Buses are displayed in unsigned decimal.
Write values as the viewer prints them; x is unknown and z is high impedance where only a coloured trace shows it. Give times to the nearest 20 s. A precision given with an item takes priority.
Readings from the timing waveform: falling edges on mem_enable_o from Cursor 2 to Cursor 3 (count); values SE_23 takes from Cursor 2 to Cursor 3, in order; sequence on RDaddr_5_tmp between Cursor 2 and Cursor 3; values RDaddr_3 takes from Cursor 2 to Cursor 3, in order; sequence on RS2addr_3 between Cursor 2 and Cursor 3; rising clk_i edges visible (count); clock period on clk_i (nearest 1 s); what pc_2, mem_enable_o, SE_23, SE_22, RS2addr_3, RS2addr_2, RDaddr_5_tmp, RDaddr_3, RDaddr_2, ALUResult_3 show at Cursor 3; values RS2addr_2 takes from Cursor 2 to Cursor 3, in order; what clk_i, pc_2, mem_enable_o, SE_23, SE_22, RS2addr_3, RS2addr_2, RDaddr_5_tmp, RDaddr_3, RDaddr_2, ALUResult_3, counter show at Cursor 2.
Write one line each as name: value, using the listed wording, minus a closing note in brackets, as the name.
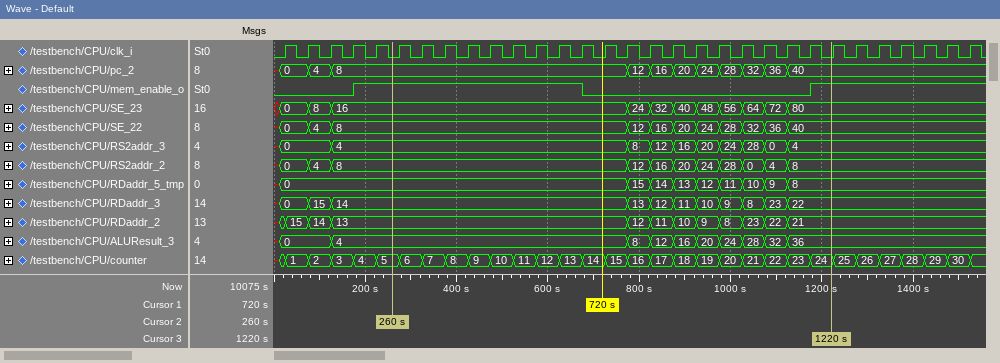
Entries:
falling edges on mem_enable_o from Cursor 2 to Cursor 3: 1
values SE_23 takes from Cursor 2 to Cursor 3, in order: 16, 24, 32, 40, 48, 56, 64, 72, 80
sequence on RDaddr_5_tmp between Cursor 2 and Cursor 3: 0, 15, 14, 13, 12, 11, 10, 9, 8
values RDaddr_3 takes from Cursor 2 to Cursor 3, in order: 14, 13, 12, 11, 10, 9, 8, 23, 22
sequence on RS2addr_3 between Cursor 2 and Cursor 3: 4, 8, 12, 16, 20, 24, 28, 0, 4
rising clk_i edges visible: 31
clock period on clk_i: 50 s
what pc_2, mem_enable_o, SE_23, SE_22, RS2addr_3, RS2addr_2, RDaddr_5_tmp, RDaddr_3, RDaddr_2, ALUResult_3 show at Cursor 3: pc_2=40, mem_enable_o=1, SE_23=80, SE_22=40, RS2addr_3=4, RS2addr_2=8, RDaddr_5_tmp=8, RDaddr_3=22, RDaddr_2=21, ALUResult_3=36
values RS2addr_2 takes from Cursor 2 to Cursor 3, in order: 8, 12, 16, 20, 24, 28, 0, 4, 8
what clk_i, pc_2, mem_enable_o, SE_23, SE_22, RS2addr_3, RS2addr_2, RDaddr_5_tmp, RDaddr_3, RDaddr_2, ALUResult_3, counter show at Cursor 2: clk_i=0, pc_2=8, mem_enable_o=1, SE_23=16, SE_22=8, RS2addr_3=4, RS2addr_2=8, RDaddr_5_tmp=0, RDaddr_3=14, RDaddr_2=13, ALUResult_3=4, counter=5
